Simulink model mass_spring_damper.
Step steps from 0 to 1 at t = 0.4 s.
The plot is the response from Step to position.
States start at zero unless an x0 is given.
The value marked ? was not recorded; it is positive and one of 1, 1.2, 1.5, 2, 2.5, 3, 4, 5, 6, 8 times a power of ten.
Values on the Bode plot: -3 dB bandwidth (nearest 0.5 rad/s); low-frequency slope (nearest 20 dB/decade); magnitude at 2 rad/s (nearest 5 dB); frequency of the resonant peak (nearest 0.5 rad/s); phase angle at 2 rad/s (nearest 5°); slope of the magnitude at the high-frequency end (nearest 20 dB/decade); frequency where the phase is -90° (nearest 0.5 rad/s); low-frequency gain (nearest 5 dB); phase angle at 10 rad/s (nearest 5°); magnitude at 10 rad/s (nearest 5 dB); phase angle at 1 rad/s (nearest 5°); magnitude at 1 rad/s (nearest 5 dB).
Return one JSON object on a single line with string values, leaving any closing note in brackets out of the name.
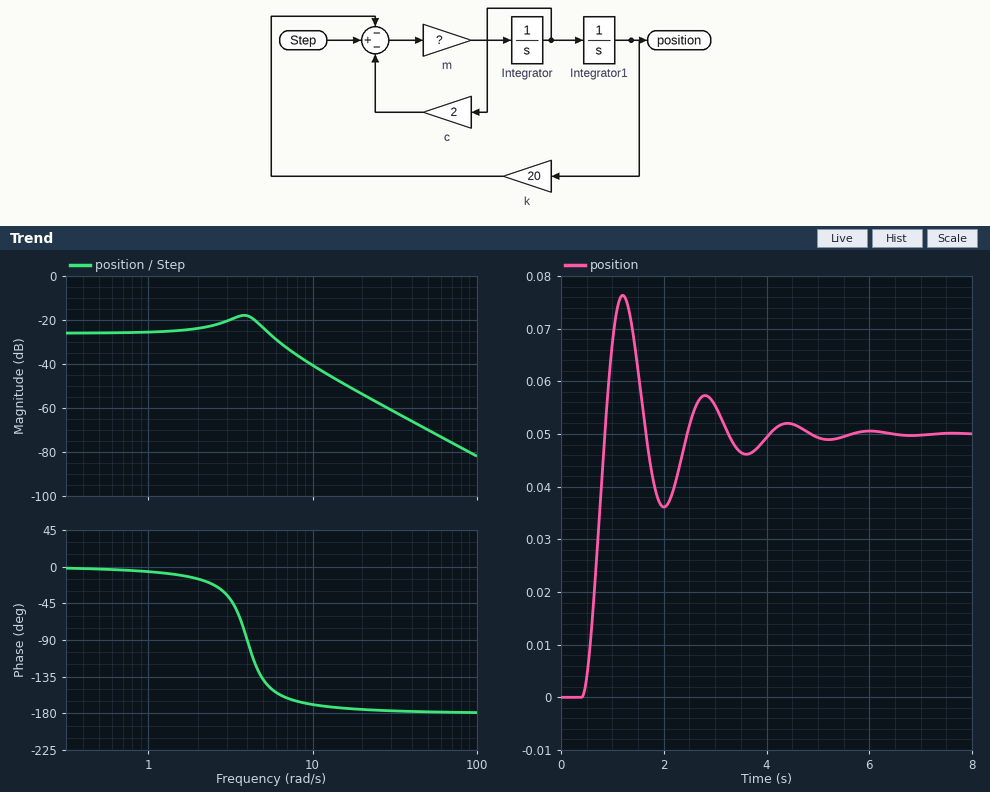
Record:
{"-3 dB bandwidth": "6.0 rad/s", "low-frequency slope": "0 dB/decade", "magnitude at 2 rad/s": "-25 dB", "frequency of the resonant peak": "4.0 rad/s", "phase angle at 2 rad/s": "-15°", "slope of the magnitude at the high-frequency end": "-40 dB/decade", "frequency where the phase is -90°": "4.0 rad/s", "low-frequency gain": "-25 dB", "phase angle at 10 rad/s": "-170°", "magnitude at 10 rad/s": "-40 dB", "phase angle at 1 rad/s": "-5°", "magnitude at 1 rad/s": "-25 dB"}
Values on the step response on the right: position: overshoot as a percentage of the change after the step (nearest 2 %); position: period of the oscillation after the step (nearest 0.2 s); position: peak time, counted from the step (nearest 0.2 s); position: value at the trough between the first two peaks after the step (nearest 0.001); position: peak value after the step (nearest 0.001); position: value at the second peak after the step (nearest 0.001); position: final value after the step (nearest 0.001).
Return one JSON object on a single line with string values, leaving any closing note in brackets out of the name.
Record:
{"position: overshoot as a percentage of the change after the step": "52 %", "position: period of the oscillation after the step": "1.6 s", "position: peak time, counted from the step": "0.8 s", "position: value at the trough between the first two peaks after the step": "0.036", "position: peak value after the step": "0.076", "position: value at the second peak after the step": "0.057", "position: final value after the step": "0.050"}
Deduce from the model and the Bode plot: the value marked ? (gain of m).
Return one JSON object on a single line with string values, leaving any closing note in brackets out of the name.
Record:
{"the value marked ?": "0.8"}
